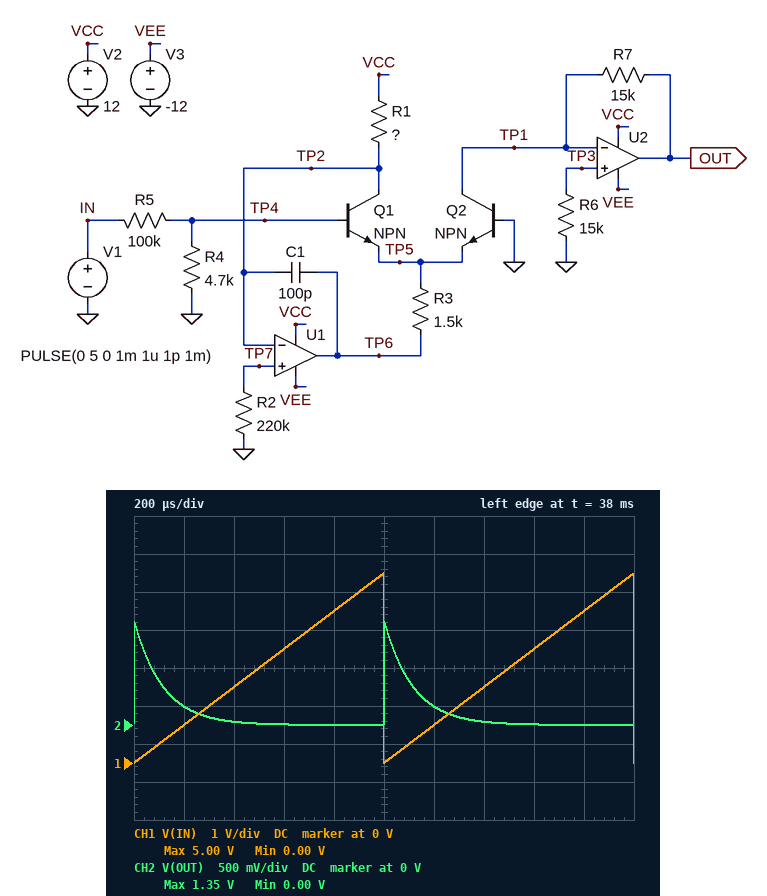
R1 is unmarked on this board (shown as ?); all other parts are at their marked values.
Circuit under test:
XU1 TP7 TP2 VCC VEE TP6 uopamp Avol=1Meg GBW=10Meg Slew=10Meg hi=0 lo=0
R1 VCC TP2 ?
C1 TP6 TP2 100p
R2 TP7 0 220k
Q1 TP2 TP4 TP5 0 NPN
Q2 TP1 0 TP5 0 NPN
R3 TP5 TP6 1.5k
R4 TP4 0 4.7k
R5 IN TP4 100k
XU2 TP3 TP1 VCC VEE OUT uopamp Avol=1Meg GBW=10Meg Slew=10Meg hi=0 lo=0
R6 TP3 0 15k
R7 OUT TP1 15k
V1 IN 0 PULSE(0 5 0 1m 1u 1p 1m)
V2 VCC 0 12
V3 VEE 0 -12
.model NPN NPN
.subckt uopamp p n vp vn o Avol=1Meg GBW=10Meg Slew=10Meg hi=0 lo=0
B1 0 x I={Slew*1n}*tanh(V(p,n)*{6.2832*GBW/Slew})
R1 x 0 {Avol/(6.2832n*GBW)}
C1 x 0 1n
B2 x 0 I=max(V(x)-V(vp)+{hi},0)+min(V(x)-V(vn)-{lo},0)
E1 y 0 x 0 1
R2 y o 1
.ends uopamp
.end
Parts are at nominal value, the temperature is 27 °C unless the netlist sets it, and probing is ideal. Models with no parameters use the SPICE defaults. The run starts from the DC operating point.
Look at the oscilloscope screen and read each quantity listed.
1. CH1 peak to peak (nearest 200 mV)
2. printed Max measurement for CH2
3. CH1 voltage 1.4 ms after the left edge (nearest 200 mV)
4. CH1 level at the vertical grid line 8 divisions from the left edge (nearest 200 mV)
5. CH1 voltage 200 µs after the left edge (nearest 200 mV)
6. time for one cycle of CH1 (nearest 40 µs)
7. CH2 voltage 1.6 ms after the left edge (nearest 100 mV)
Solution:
5.0 V
1.35 V
2.0 V
3.0 V
1.0 V
1.00 ms
0 V
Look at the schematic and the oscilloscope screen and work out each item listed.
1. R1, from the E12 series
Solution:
150 kΩ
